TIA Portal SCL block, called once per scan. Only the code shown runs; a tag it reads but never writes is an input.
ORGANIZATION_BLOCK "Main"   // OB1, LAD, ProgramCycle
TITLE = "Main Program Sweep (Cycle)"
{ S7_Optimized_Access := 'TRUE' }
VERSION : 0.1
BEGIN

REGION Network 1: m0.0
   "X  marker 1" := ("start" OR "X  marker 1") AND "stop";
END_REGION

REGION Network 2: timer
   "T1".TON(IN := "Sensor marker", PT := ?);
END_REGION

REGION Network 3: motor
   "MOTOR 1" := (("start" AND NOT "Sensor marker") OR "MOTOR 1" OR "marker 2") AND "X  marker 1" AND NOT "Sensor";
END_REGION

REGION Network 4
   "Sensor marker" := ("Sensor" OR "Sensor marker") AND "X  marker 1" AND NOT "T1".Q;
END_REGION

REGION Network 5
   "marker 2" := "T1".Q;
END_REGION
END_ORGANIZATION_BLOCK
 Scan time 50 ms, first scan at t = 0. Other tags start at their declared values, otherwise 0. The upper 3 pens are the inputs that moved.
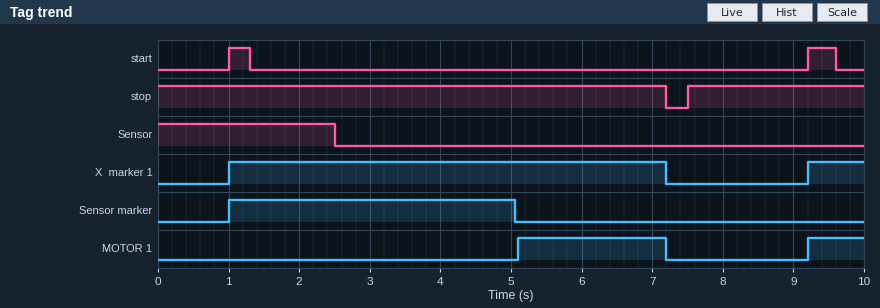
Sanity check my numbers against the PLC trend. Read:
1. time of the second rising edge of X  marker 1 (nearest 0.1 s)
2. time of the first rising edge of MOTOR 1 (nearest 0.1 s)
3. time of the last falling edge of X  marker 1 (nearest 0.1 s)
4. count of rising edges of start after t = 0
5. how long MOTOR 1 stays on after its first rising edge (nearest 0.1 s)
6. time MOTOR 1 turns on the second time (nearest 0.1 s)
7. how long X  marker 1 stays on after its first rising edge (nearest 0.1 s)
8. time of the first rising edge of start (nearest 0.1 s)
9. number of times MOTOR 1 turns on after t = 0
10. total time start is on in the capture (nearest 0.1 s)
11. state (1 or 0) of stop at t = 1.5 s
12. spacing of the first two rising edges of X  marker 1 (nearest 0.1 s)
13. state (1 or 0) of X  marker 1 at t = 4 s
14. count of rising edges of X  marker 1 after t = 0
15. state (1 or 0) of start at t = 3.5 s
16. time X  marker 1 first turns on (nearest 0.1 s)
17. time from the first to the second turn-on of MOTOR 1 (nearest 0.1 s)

9.2 s
5.1 s
7.2 s
2
2.1 s
9.2 s
6.2 s
1.0 s
2
0.7 s
1
8.2 s
1
2
0
1.0 s
4.1 s
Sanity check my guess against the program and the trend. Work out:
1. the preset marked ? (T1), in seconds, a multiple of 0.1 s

4.0 s
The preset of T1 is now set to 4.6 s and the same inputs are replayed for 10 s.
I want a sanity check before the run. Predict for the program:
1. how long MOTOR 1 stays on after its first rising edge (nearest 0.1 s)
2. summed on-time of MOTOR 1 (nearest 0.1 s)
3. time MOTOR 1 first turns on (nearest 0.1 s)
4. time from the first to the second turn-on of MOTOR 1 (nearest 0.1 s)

1.5 s
2.3 s
5.7 s
3.5 s
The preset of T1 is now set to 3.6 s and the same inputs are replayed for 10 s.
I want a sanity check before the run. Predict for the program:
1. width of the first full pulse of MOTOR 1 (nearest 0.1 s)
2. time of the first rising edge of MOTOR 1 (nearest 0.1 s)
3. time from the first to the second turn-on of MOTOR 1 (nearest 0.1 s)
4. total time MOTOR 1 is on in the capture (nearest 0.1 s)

2.5 s
4.7 s
4.5 s
3.3 s
